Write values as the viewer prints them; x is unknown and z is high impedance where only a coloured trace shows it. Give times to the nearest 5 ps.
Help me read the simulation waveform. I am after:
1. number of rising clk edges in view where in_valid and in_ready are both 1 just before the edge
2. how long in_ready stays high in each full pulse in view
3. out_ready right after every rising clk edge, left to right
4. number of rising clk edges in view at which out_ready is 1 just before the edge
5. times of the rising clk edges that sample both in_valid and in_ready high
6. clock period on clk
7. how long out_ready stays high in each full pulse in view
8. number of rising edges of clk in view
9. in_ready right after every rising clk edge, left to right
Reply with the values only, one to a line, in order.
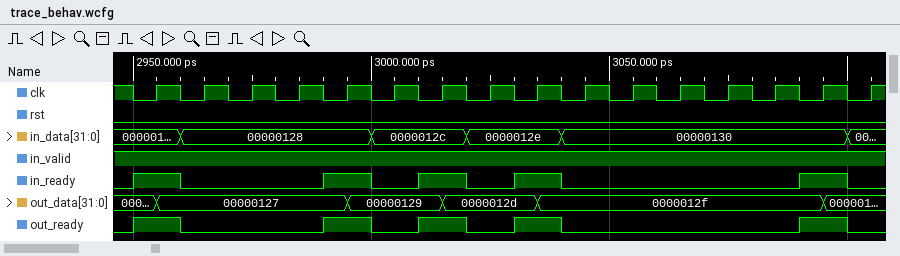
5
10 ps, 10 ps, 10 ps, 10 ps, 10 ps
1 0 0 0 1 0 1 0 1 0 0 0 0 0 1 0
5
2955 ps, 2995 ps, 3015 ps, 3035 ps, 3095 ps
10 ps
10 ps, 10 ps, 10 ps, 10 ps, 10 ps
16
1 0 0 0 1 0 1 0 1 0 0 0 0 0 1 0
